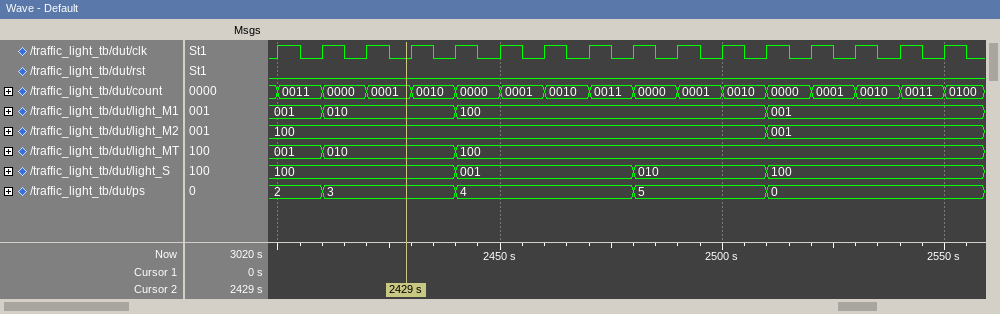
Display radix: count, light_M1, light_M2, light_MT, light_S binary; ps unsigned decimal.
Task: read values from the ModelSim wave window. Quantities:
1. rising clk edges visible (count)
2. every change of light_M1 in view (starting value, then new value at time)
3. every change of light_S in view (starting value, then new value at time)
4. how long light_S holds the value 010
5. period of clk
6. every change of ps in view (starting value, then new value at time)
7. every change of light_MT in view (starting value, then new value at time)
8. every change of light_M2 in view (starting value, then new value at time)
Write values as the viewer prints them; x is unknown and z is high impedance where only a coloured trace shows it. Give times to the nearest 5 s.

16
001, 010 at 2410 s, 100 at 2440 s, 001 at 2510 s
100, 001 at 2440 s, 010 at 2480 s, 100 at 2510 s
30 s
10 s
2, 3 at 2410 s, 4 at 2440 s, 5 at 2480 s, 0 at 2510 s
001, 010 at 2410 s, 100 at 2440 s
100, 001 at 2510 s
